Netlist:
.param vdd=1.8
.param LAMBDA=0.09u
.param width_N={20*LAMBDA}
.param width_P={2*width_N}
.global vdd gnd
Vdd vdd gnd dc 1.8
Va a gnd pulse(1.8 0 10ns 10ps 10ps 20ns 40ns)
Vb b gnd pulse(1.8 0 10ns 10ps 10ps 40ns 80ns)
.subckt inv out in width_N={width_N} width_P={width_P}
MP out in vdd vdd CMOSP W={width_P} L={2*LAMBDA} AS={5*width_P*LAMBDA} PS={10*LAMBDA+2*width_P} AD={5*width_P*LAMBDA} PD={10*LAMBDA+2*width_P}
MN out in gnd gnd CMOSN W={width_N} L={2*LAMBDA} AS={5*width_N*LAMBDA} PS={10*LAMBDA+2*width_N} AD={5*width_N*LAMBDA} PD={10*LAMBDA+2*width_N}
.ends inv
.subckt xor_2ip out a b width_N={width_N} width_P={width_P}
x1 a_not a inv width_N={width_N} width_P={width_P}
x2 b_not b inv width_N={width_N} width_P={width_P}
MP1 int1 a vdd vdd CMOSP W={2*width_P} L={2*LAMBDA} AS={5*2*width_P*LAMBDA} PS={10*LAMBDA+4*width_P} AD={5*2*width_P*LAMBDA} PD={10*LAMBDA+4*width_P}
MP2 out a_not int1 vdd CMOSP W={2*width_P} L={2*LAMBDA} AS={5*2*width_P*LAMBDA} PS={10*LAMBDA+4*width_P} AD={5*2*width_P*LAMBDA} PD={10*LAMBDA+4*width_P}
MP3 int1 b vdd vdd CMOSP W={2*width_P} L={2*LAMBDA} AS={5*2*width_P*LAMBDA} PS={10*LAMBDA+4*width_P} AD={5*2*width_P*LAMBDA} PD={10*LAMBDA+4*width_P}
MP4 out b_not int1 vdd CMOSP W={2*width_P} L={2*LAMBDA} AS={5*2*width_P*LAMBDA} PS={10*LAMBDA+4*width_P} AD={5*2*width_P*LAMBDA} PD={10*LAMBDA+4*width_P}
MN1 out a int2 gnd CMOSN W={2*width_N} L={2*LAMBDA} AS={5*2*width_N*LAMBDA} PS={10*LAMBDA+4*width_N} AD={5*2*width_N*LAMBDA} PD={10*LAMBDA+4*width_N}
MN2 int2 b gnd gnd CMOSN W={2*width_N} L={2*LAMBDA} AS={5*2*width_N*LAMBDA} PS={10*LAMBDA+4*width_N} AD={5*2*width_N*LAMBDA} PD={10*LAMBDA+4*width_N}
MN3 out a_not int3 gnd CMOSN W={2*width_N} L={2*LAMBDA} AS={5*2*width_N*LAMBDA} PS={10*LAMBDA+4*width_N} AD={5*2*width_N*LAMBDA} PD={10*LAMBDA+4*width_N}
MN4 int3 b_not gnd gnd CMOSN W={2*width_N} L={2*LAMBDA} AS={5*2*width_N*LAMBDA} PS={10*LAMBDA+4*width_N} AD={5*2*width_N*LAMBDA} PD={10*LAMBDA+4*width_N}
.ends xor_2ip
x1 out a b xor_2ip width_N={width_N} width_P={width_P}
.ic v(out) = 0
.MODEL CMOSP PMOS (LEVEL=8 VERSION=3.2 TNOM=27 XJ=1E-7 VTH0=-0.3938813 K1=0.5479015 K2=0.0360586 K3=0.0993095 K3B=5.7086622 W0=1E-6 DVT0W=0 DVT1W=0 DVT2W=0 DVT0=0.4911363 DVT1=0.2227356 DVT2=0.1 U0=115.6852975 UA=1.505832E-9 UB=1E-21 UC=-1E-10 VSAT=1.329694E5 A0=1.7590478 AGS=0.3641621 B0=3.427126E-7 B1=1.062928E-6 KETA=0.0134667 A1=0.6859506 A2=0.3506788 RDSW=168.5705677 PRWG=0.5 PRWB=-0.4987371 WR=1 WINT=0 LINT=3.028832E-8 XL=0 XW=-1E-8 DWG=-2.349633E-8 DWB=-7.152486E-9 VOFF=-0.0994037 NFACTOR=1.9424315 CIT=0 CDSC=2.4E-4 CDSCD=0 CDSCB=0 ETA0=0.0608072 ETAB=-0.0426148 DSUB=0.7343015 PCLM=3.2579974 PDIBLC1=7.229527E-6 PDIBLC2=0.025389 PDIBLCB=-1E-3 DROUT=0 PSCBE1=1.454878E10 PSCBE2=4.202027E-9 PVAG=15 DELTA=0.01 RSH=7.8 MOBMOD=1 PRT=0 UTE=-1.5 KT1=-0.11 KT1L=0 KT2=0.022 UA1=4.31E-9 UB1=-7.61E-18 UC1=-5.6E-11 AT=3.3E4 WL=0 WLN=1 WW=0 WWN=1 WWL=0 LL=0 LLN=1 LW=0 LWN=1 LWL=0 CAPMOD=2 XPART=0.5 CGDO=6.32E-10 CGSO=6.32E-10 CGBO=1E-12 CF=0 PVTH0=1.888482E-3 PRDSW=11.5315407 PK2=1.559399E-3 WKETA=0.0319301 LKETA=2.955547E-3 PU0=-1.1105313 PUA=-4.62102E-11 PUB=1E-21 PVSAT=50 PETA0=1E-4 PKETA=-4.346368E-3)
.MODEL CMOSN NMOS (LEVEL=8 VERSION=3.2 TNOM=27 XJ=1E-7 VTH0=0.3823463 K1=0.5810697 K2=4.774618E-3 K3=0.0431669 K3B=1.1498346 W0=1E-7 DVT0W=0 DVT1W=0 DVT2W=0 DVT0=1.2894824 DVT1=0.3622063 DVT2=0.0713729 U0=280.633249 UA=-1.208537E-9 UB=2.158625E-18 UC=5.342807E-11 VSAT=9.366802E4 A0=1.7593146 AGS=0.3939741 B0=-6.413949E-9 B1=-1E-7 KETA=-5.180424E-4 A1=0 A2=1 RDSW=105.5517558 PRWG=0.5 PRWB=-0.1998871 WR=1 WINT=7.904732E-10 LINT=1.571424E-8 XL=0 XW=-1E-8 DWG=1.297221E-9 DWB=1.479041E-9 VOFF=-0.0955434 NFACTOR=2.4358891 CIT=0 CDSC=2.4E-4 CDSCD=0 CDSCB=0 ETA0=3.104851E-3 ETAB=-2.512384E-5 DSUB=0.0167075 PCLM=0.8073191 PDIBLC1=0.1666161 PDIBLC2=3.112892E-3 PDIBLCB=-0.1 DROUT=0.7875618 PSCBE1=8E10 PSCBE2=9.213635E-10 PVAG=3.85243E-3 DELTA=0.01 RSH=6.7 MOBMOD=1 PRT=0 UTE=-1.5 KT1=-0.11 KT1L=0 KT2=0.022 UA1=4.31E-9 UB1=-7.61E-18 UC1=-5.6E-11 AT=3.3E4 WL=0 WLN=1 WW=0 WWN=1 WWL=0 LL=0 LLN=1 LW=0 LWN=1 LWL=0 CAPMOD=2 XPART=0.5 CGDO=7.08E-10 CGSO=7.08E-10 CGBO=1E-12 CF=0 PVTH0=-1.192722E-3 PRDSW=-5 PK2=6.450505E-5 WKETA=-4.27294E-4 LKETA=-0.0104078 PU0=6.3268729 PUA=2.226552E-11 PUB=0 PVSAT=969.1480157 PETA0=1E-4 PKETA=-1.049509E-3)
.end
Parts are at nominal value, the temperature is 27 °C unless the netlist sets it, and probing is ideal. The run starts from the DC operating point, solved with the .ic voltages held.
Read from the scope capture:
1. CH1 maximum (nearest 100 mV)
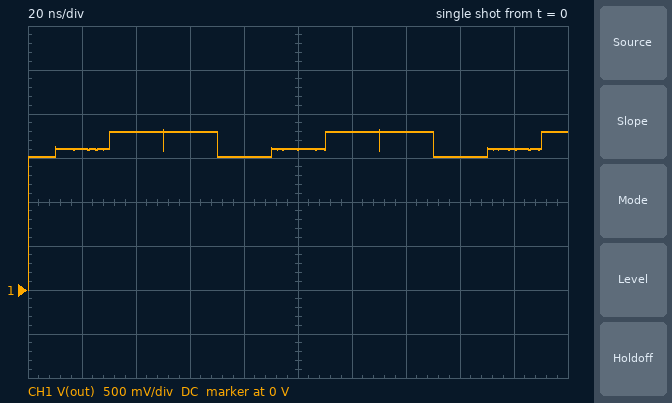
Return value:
1.8 V
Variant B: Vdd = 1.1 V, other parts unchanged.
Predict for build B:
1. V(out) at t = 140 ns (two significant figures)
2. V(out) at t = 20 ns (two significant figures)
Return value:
1.1 V
1.0 V
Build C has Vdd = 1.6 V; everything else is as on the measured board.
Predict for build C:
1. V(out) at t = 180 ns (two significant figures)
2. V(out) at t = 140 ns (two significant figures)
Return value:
1.4 V
1.6 V
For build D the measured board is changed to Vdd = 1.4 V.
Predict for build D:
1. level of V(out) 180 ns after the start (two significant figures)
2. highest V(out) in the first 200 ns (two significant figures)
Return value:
1.3 V
1.4 V
